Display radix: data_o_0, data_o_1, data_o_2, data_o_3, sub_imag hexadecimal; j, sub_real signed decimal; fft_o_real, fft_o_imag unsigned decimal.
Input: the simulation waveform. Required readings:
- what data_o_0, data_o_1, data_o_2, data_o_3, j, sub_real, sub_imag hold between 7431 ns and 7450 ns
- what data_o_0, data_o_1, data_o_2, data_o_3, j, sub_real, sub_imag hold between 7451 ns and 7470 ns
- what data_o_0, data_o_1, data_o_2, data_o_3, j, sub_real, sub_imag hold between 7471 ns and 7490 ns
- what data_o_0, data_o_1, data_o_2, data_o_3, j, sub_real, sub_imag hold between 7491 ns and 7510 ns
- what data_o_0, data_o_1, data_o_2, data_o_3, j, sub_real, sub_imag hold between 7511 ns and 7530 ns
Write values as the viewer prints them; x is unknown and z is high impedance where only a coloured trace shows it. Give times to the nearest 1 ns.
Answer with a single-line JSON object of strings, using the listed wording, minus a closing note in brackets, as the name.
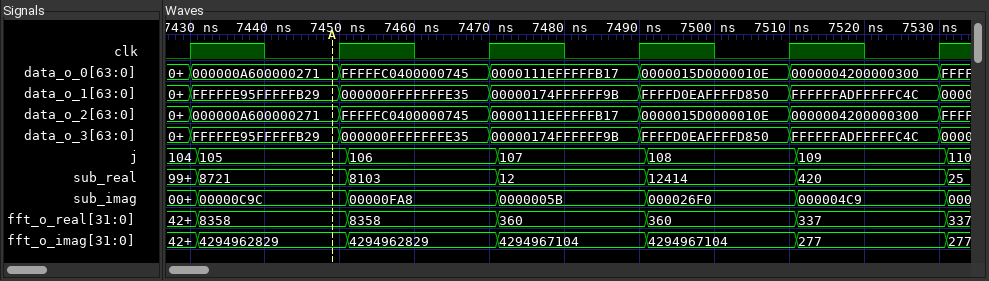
{"what data_o_0, data_o_1, data_o_2, data_o_3, j, sub_real, sub_imag hold between 7431 ns and 7450 ns": "data_o_0=000000A600000271, data_o_1=FFFFFE95FFFFFB29, data_o_2=000000A600000271, data_o_3=FFFFFE95FFFFFB29, j=105, sub_real=8721, sub_imag=00000C9C", "what data_o_0, data_o_1, data_o_2, data_o_3, j, sub_real, sub_imag hold between 7451 ns and 7470 ns": "data_o_0=FFFFFC0400000745, data_o_1=000000FFFFFFFE35, data_o_2=FFFFFC0400000745, data_o_3=000000FFFFFFFE35, j=106, sub_real=8103, sub_imag=00000FA8", "what data_o_0, data_o_1, data_o_2, data_o_3, j, sub_real, sub_imag hold between 7471 ns and 7490 ns": "data_o_0=0000111EFFFFFB17, data_o_1=00000174FFFFFF9B, data_o_2=0000111EFFFFFB17, data_o_3=00000174FFFFFF9B, j=107, sub_real=12, sub_imag=0000005B", "what data_o_0, data_o_1, data_o_2, data_o_3, j, sub_real, sub_imag hold between 7491 ns and 7510 ns": "data_o_0=0000015D0000010E, data_o_1=FFFFD0EAFFFFD850, data_o_2=0000015D0000010E, data_o_3=FFFFD0EAFFFFD850, j=108, sub_real=12414, sub_imag=000026F0", "what data_o_0, data_o_1, data_o_2, data_o_3, j, sub_real, sub_imag hold between 7511 ns and 7530 ns": "data_o_0=0000004200000300, data_o_1=FFFFFFADFFFFFC4C, data_o_2=0000004200000300, data_o_3=FFFFFFADFFFFFC4C, j=109, sub_real=420, sub_imag=000004C9"}
